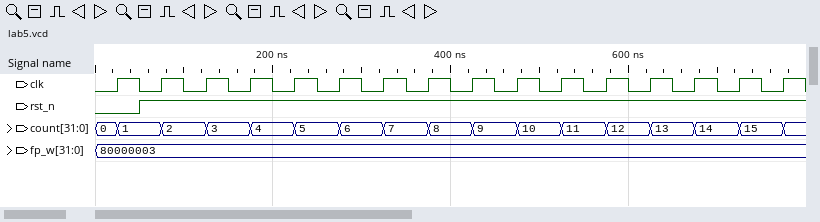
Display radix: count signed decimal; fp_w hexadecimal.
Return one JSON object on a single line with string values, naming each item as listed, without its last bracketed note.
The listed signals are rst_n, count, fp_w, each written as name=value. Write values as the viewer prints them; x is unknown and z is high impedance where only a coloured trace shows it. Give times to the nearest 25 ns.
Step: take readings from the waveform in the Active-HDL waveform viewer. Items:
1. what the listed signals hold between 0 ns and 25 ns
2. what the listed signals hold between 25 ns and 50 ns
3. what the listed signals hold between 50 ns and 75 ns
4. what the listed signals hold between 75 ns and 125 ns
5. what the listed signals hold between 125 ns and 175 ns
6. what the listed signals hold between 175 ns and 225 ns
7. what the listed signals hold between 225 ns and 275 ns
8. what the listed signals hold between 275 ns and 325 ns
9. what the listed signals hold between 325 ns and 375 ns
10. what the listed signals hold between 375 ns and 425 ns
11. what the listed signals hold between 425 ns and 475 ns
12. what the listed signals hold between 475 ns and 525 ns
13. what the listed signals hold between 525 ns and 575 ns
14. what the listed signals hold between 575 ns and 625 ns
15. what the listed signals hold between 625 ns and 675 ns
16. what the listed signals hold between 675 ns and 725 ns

{"what the listed signals hold between 0 ns and 25 ns": "rst_n=0, count=0, fp_w=80000003", "what the listed signals hold between 25 ns and 50 ns": "rst_n=0, count=1, fp_w=80000003", "what the listed signals hold between 50 ns and 75 ns": "rst_n=1, count=1, fp_w=80000003", "what the listed signals hold between 75 ns and 125 ns": "rst_n=1, count=2, fp_w=80000003", "what the listed signals hold between 125 ns and 175 ns": "rst_n=1, count=3, fp_w=80000003", "what the listed signals hold between 175 ns and 225 ns": "rst_n=1, count=4, fp_w=80000003", "what the listed signals hold between 225 ns and 275 ns": "rst_n=1, count=5, fp_w=80000003", "what the listed signals hold between 275 ns and 325 ns": "rst_n=1, count=6, fp_w=80000003", "what the listed signals hold between 325 ns and 375 ns": "rst_n=1, count=7, fp_w=80000003", "what the listed signals hold between 375 ns and 425 ns": "rst_n=1, count=8, fp_w=80000003", "what the listed signals hold between 425 ns and 475 ns": "rst_n=1, count=9, fp_w=80000003", "what the listed signals hold between 475 ns and 525 ns": "rst_n=1, count=10, fp_w=80000003", "what the listed signals hold between 525 ns and 575 ns": "rst_n=1, count=11, fp_w=80000003", "what the listed signals hold between 575 ns and 625 ns": "rst_n=1, count=12, fp_w=80000003", "what the listed signals hold between 625 ns and 675 ns": "rst_n=1, count=13, fp_w=80000003", "what the listed signals hold between 675 ns and 725 ns": "rst_n=1, count=14, fp_w=80000003"}
